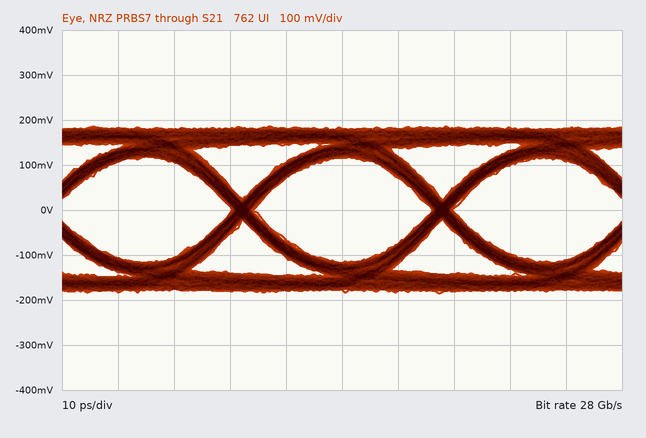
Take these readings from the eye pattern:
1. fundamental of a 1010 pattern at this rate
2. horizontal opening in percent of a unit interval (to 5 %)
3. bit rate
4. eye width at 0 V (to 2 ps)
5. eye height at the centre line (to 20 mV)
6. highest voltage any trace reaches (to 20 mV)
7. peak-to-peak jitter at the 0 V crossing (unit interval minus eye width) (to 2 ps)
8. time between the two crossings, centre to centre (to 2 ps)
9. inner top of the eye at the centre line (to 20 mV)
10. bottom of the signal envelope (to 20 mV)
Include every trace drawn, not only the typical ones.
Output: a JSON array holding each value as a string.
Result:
["14 GHz", "90 %", "28 Gb/s", "32 ps", "240 mV", "180 mV", "4 ps", "36 ps", "120 mV", "-180 mV"]
